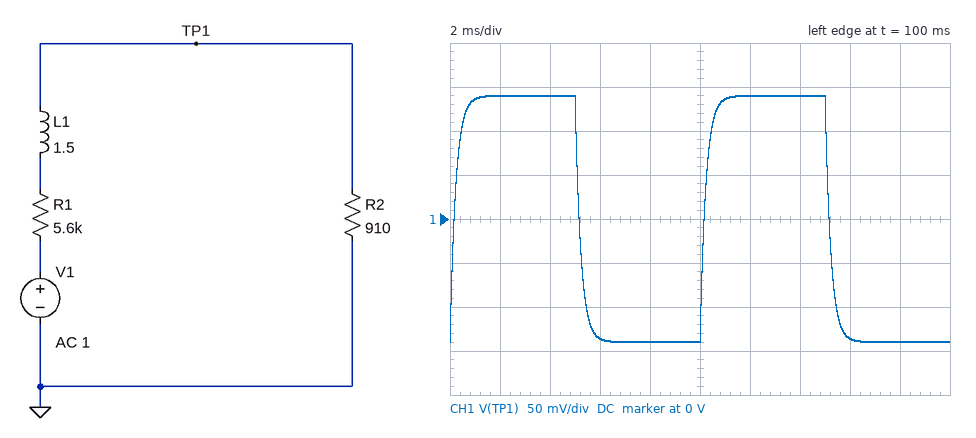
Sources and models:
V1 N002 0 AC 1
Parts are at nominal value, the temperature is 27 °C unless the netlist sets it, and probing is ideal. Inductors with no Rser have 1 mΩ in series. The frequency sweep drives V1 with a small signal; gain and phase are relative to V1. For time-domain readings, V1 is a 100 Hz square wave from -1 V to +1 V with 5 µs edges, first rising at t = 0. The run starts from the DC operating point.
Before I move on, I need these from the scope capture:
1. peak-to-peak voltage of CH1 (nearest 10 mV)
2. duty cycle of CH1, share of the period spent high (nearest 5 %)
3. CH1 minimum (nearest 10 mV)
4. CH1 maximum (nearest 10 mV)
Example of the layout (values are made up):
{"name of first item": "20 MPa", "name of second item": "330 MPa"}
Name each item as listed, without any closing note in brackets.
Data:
{"peak-to-peak voltage of CH1": "280 mV", "duty cycle of CH1, share of the period spent high": "50 %", "CH1 minimum": "-140 mV", "CH1 maximum": "140 mV"}
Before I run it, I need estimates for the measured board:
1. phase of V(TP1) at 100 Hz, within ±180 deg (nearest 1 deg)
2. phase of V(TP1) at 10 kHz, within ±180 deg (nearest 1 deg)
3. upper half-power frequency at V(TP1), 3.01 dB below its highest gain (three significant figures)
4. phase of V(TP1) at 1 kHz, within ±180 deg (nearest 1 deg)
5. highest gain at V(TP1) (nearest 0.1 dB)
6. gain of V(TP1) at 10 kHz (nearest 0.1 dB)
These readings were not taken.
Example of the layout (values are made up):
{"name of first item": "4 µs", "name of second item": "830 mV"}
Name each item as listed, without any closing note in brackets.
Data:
{"phase of V(TP1) at 100 Hz, within ±180 deg": "-8 deg", "phase of V(TP1) at 10 kHz, within ±180 deg": "-86 deg", "upper half-power frequency at V(TP1), 3.01 dB below its highest gain": "691 Hz", "phase of V(TP1) at 1 kHz, within ±180 deg": "-55 deg", "highest gain at V(TP1)": "-17.1 dB", "gain of V(TP1) at 10 kHz": "-40.3 dB"}
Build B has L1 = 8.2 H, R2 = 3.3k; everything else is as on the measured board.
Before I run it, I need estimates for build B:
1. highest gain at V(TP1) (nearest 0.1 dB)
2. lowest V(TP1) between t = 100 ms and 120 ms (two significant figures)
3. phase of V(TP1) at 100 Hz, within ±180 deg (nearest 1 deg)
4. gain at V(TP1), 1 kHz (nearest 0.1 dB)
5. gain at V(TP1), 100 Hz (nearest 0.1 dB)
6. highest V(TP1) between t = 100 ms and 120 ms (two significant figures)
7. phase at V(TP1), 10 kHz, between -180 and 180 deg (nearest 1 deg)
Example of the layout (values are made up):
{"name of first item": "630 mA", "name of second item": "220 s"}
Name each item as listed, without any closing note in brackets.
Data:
{"highest gain at V(TP1)": "-8.6 dB", "lowest V(TP1) between t = 100 ms and 120 ms": "-370 mV", "phase of V(TP1) at 100 Hz, within ±180 deg": "-30 deg", "gain at V(TP1), 1 kHz": "-24.0 dB", "gain at V(TP1), 100 Hz": "-9.9 dB", "highest V(TP1) between t = 100 ms and 120 ms": "370 mV", "phase at V(TP1), 10 kHz, between -180 and 180 deg": "-89 deg"}
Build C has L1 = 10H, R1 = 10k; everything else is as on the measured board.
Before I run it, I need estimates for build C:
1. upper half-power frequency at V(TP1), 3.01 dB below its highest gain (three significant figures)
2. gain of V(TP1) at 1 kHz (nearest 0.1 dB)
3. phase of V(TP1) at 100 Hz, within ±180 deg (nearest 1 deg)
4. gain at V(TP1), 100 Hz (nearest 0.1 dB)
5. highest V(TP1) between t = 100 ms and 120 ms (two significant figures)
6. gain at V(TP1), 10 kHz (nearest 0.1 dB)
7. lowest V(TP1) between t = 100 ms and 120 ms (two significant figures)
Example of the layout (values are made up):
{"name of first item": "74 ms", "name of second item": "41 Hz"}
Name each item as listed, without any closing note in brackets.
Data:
{"upper half-power frequency at V(TP1), 3.01 dB below its highest gain": "174 Hz", "gain of V(TP1) at 1 kHz": "-36.9 dB", "phase of V(TP1) at 100 Hz, within ±180 deg": "-30 deg", "gain at V(TP1), 100 Hz": "-22.8 dB", "highest V(TP1) between t = 100 ms and 120 ms": "83 mV", "gain at V(TP1), 10 kHz": "-56.8 dB", "lowest V(TP1) between t = 100 ms and 120 ms": "-83 mV"}
